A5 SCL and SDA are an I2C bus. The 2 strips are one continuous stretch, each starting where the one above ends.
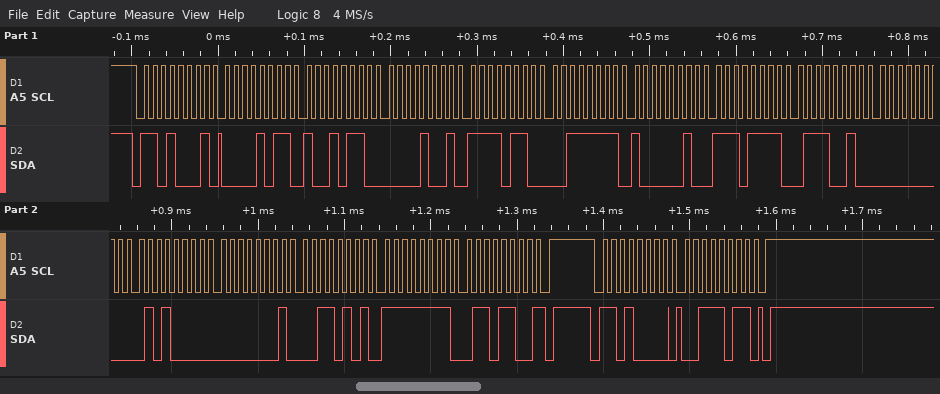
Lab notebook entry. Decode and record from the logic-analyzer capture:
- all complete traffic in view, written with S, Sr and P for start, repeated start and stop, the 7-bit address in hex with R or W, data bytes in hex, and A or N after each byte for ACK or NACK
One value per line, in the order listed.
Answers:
S 68R A 0B A 96 A 09 A F6 A 3F A 82 A EF A 72 A 00 A 50 A 01 A 35 A FF A 6C N P S 68W A 3B A P
